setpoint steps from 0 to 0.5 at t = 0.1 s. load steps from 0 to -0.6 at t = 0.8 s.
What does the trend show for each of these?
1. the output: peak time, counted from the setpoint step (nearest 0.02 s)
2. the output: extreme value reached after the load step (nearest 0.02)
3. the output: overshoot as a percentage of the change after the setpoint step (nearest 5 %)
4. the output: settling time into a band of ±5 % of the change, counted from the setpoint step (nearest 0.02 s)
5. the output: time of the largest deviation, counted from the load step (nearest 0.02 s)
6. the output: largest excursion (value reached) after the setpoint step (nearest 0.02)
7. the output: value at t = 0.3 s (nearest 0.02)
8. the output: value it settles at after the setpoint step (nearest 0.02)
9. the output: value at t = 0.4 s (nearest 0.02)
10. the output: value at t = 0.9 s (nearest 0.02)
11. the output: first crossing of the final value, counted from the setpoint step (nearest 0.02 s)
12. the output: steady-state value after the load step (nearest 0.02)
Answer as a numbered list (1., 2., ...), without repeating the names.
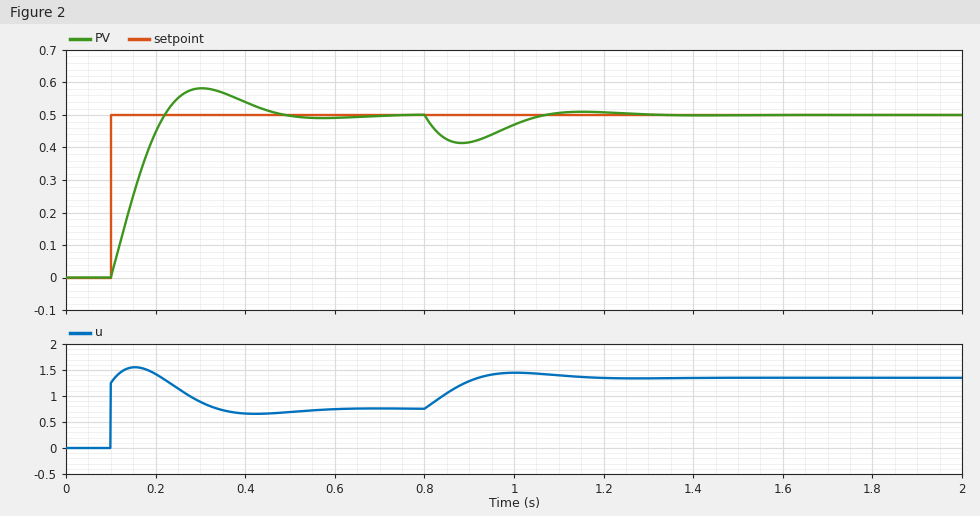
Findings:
1. 0.20 s
2. 0.42
3. 15 %
4. 0.32 s
5. 0.08 s
6. 0.58
7. 0.58
8. 0.50
9. 0.54
10. 0.42
11. 0.12 s
12. 0.50
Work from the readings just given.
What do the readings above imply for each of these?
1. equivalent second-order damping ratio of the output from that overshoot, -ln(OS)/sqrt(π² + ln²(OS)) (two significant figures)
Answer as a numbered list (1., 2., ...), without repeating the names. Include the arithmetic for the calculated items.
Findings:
1. ln(0.15) = -1.897; 1.897 / sqrt(9.870 + 3.599) = 0.52
